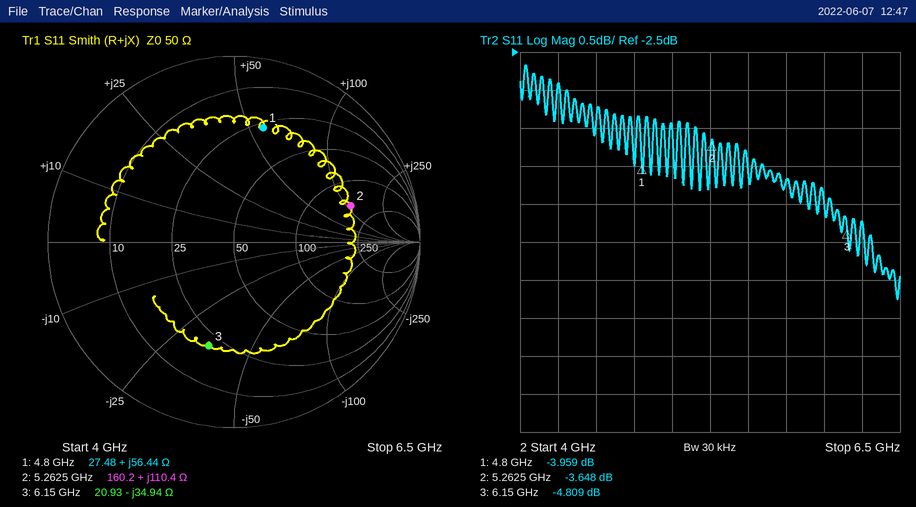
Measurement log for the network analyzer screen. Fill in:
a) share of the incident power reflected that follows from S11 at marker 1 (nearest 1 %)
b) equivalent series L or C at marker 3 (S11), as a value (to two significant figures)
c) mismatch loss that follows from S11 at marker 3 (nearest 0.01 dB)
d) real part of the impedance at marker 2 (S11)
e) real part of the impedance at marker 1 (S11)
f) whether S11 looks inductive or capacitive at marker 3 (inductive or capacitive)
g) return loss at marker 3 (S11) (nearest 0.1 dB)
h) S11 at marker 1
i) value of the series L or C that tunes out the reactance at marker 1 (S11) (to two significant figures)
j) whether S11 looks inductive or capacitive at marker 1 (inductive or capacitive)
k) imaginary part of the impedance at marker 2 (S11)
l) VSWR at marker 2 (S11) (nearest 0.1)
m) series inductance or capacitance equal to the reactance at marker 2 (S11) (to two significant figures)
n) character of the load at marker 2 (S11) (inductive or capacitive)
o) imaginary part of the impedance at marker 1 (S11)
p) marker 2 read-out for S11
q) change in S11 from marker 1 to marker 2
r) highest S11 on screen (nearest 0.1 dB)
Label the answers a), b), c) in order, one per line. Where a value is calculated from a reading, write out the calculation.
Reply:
a) 10^(-3.959/10) ≈ 40 %
b) C = 1/(2π × 6.15 GHz × 34.94 Ω) ≈ 741 fF, so 740 fF to two significant figures
c) −10 log10(1 − 10^(-4.809/10)) ≈ 1.74 dB
d) 160.2 Ω
e) 27.48 Ω
f) capacitive
g) 4.8 dB
h) -3.959 dB
i) C = 1/(2π × 4.8 GHz × 56.44 Ω) ≈ 587 fF, so 590 fF to two significant figures
j) inductive
k) +110.4 Ω
l) (1 + 0.6571)/(1 − 0.6571) ≈ 4.8
m) L = 110.4 Ω/(2π × 5.2625 GHz) ≈ 3.3 nH
n) inductive
o) +56.44 Ω
p) -3.648 dB
q) -3.648 − (-3.959) = 0.311 dB
r) -2.7 dB
